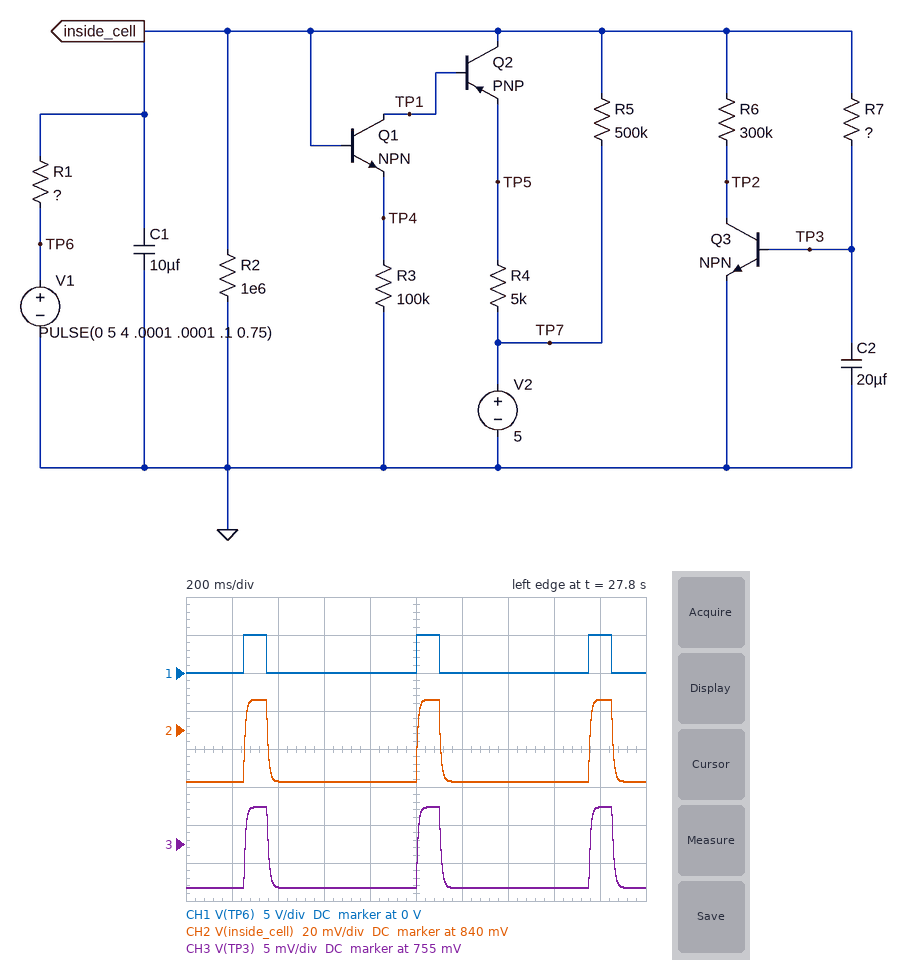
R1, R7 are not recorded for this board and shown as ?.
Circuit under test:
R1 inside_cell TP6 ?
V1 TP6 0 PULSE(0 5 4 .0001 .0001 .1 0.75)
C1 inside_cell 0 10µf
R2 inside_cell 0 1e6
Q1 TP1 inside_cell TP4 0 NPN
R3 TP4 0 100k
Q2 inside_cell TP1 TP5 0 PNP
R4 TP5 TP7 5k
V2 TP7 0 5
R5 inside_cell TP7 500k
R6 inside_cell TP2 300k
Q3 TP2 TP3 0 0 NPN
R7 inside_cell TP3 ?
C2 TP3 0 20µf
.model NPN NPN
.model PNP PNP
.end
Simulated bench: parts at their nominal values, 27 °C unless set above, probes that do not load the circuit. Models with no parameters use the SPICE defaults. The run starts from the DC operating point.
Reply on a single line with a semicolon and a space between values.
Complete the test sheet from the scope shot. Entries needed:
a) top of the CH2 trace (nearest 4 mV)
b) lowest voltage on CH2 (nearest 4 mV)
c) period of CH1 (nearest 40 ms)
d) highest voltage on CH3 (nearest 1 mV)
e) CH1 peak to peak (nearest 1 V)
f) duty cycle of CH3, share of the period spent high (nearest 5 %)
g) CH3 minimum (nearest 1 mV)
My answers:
856 mV; 812 mV; 760 ms; 760 mV; 5 V; 15 %; 749 mV
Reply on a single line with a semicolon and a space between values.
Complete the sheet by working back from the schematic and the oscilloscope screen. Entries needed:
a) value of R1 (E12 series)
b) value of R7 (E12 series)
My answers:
82 kΩ; 330 Ω
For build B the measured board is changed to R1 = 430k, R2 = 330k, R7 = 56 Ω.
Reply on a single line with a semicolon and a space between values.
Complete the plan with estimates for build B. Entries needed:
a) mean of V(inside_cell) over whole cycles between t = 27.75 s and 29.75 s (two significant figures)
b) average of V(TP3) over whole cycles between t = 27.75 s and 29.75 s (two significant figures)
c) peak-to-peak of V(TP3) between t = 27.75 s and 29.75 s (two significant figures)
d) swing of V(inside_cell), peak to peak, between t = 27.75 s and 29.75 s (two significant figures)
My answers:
750 mV; 740 mV; 2.4 mV; 3.2 mV
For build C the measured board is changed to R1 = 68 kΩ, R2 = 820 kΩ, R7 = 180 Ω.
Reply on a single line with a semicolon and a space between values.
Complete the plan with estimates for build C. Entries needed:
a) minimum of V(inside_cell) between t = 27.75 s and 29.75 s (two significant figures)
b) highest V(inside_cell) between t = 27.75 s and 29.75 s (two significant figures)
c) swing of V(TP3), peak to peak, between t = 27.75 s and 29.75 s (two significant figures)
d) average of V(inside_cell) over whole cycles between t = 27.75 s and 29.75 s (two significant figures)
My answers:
770 mV; 800 mV; 13 mV; 780 mV
